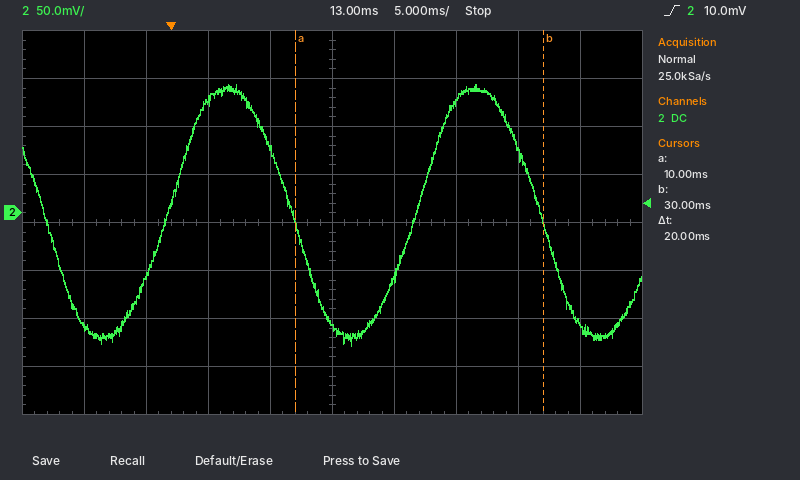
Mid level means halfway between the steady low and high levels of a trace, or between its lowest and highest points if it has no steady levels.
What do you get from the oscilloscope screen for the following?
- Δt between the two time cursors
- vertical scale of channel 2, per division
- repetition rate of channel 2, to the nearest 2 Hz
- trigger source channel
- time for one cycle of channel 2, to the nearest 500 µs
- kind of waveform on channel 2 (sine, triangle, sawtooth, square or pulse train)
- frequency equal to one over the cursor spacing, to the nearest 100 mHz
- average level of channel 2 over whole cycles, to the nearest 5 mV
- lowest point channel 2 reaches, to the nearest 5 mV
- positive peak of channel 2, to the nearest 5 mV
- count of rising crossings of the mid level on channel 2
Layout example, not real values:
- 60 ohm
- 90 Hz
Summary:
- 20 ms
- 50 mV
- 50 Hz
- channel 2
- 20.0 ms
- sine
- 50.0 Hz
- 0 mV
- -140 mV
- 135 mV
- 2
